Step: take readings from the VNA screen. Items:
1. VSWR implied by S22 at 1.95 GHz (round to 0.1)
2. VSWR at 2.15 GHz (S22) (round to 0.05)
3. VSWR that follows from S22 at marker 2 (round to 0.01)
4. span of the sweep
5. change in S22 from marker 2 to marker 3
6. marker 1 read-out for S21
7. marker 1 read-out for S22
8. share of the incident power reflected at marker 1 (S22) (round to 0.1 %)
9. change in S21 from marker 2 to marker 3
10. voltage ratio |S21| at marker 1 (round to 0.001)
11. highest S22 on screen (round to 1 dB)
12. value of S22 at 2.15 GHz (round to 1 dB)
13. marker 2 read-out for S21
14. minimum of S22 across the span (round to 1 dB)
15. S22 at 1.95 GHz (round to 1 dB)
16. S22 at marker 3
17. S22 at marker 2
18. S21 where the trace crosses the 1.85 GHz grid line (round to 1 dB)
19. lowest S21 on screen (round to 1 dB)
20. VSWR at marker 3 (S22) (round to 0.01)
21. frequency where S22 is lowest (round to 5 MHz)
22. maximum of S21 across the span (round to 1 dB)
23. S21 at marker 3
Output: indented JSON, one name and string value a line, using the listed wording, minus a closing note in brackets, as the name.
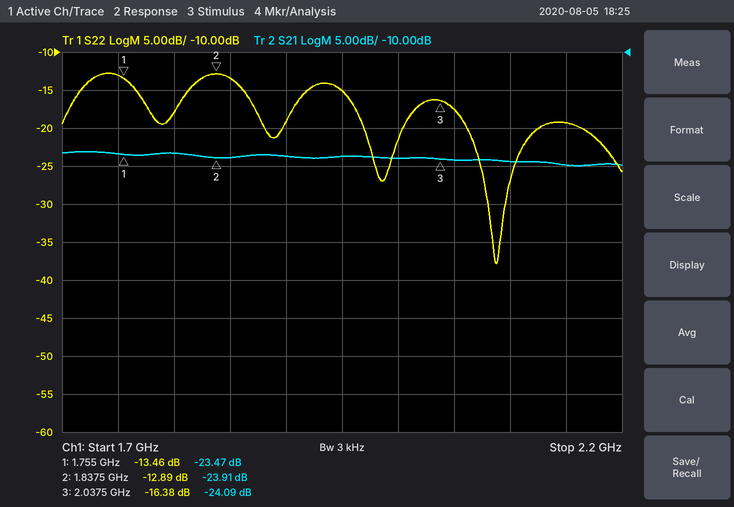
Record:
{
  "VSWR implied by S22 at 1.95 GHz": "1.4",
  "VSWR at 2.15 GHz (S22)": "1.25",
  "VSWR that follows from S22 at marker 2": "1.59",
  "span of the sweep": "500 MHz",
  "change in S22 from marker 2 to marker 3": "-3.49 dB",
  "marker 1 read-out for S21": "-23.47 dB",
  "marker 1 read-out for S22": "-13.46 dB",
  "share of the incident power reflected at marker 1 (S22)": "4.5 %",
  "change in S21 from marker 2 to marker 3": "-0.18 dB",
  "voltage ratio |S21| at marker 1": "0.067",
  "highest S22 on screen": "-13 dB",
  "value of S22 at 2.15 GHz": "-19 dB",
  "marker 2 read-out for S21": "-23.91 dB",
  "minimum of S22 across the span": "-38 dB",
  "S22 at 1.95 GHz": "-15 dB",
  "S22 at marker 3": "-16.38 dB",
  "S22 at marker 2": "-12.89 dB",
  "S21 where the trace crosses the 1.85 GHz grid line": "-24 dB",
  "lowest S21 on screen": "-25 dB",
  "VSWR at marker 3 (S22)": "1.36",
  "frequency where S22 is lowest": "2.090 GHz",
  "maximum of S21 across the span": "-23 dB",
  "S21 at marker 3": "-24.09 dB"
}
